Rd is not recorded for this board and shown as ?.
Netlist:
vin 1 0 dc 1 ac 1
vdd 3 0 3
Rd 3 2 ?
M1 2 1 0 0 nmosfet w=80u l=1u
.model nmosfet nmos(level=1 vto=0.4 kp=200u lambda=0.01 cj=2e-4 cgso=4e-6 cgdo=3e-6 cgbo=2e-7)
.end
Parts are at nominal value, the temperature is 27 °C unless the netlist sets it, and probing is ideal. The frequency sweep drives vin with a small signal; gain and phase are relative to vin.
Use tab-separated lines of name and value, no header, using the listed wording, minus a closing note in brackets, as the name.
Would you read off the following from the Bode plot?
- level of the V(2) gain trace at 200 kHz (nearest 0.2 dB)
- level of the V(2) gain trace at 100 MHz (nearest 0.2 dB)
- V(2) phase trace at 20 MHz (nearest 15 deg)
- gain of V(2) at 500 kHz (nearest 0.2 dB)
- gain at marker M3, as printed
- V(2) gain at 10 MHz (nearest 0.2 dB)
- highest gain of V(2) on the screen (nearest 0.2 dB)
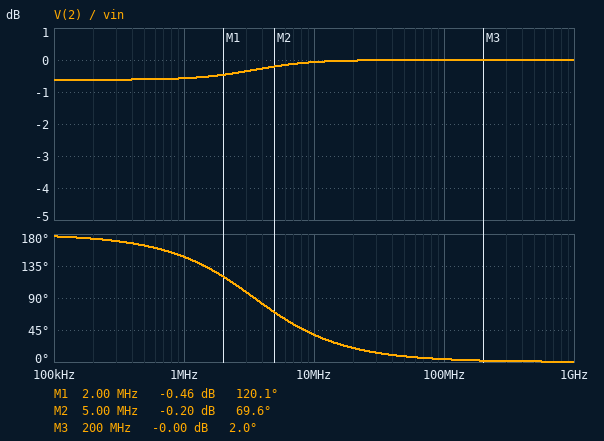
level of the V(2) gain trace at 200 kHz	-0.6 dB
level of the V(2) gain trace at 100 MHz	0 dB
V(2) phase trace at 20 MHz	15 deg
gain of V(2) at 500 kHz	-0.6 dB
gain at marker M3, as printed	-0.00 dB
V(2) gain at 10 MHz	0 dB
highest gain of V(2) on the screen	0 dB
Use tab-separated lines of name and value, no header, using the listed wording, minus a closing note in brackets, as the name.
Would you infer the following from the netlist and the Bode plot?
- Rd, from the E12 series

Rd, from the E12 series	1.2 kΩ
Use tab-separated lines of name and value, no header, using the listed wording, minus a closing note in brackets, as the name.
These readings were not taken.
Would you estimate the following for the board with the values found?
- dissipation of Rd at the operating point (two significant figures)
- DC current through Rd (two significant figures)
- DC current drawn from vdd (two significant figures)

dissipation of Rd at the operating point	6.0 mW
DC current through Rd	2.2 mA
DC current drawn from vdd	2.2 mA
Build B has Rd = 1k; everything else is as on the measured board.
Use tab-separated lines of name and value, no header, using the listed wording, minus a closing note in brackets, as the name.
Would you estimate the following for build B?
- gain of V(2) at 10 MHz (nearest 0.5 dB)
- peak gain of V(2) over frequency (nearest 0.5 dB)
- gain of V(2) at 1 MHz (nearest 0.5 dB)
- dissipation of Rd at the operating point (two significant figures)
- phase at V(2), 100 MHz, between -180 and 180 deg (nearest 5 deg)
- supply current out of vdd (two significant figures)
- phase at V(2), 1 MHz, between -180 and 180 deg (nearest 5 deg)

gain of V(2) at 10 MHz	0.5 dB
peak gain of V(2) over frequency	4.0 dB
gain of V(2) at 1 MHz	3.5 dB
dissipation of Rd at the operating point	6.7 mW
phase at V(2), 100 MHz, between -180 and 180 deg	5 deg
supply current out of vdd	2.6 mA
phase at V(2), 1 MHz, between -180 and 180 deg	145 deg
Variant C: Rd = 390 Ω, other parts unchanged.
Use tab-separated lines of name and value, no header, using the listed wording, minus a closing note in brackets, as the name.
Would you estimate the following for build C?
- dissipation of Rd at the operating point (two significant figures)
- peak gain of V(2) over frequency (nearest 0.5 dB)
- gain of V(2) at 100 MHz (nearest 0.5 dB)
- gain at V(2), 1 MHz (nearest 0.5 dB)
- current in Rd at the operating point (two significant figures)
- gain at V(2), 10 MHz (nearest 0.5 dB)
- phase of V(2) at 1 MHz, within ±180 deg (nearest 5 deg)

dissipation of Rd at the operating point	3.4 mW
peak gain of V(2) over frequency	11.5 dB
gain of V(2) at 100 MHz	0 dB
gain at V(2), 1 MHz	10.5 dB
current in Rd at the operating point	2.9 mA
gain at V(2), 10 MHz	1.5 dB
phase of V(2) at 1 MHz, within ±180 deg	140 deg
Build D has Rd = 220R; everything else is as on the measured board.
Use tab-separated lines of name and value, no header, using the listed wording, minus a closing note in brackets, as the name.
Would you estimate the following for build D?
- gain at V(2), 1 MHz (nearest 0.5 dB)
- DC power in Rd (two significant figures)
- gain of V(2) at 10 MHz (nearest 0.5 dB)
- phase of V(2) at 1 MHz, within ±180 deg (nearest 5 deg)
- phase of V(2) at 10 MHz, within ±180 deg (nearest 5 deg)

gain at V(2), 1 MHz	6.5 dB
DC power in Rd	1.9 mW
gain of V(2) at 10 MHz	1.0 dB
phase of V(2) at 1 MHz, within ±180 deg	155 deg
phase of V(2) at 10 MHz, within ±180 deg	50 deg
